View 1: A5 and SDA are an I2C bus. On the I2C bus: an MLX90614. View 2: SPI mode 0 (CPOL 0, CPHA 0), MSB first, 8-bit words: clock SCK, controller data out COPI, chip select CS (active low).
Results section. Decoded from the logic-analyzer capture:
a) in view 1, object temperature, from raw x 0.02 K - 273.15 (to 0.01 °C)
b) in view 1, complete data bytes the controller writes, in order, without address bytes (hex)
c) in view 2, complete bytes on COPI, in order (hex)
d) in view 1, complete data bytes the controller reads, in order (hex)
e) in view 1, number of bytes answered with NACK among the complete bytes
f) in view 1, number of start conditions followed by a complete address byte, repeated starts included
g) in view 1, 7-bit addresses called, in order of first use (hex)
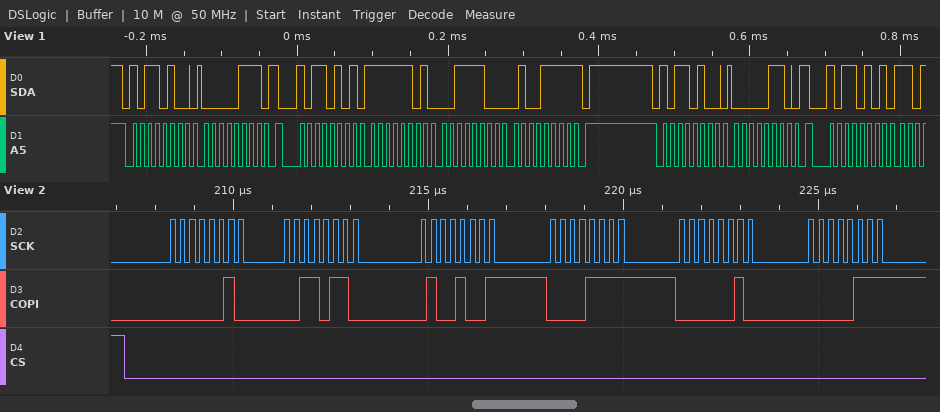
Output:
39.11 °C
07 06
02 36 49 0F 02 07
FD 3C 4F
1
4
0x5A
